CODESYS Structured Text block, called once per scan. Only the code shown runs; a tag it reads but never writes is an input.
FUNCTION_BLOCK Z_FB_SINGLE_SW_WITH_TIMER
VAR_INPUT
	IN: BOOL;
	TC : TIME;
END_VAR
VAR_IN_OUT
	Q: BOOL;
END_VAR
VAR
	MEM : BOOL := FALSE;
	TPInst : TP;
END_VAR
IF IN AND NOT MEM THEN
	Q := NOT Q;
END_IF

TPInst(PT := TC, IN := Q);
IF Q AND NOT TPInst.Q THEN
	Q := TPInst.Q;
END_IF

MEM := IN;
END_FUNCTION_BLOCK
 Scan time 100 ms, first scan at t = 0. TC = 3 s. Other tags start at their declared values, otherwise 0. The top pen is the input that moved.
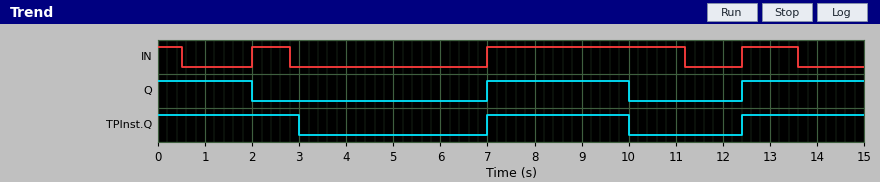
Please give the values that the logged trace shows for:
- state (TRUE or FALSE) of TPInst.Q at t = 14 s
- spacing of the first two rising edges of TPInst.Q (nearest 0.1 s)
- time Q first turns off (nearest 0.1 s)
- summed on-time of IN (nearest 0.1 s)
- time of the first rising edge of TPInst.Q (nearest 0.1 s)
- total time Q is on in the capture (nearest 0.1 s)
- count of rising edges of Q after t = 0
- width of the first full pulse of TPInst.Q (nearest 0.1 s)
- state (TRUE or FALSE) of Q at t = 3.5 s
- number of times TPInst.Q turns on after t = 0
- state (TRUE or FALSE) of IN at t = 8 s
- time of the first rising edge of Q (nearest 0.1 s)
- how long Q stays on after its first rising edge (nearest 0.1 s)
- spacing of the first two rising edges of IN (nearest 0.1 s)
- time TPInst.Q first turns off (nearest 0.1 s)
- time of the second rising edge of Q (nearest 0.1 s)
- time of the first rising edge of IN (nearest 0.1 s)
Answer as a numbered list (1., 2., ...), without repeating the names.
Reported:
1. TRUE
2. 5.4 s
3. 2.0 s
4. 6.7 s
5. 7.0 s
6. 7.6 s
7. 2
8. 3.0 s
9. FALSE
10. 2
11. TRUE
12. 7.0 s
13. 3.0 s
14. 5.0 s
15. 3.0 s
16. 12.4 s
17. 2.0 s
